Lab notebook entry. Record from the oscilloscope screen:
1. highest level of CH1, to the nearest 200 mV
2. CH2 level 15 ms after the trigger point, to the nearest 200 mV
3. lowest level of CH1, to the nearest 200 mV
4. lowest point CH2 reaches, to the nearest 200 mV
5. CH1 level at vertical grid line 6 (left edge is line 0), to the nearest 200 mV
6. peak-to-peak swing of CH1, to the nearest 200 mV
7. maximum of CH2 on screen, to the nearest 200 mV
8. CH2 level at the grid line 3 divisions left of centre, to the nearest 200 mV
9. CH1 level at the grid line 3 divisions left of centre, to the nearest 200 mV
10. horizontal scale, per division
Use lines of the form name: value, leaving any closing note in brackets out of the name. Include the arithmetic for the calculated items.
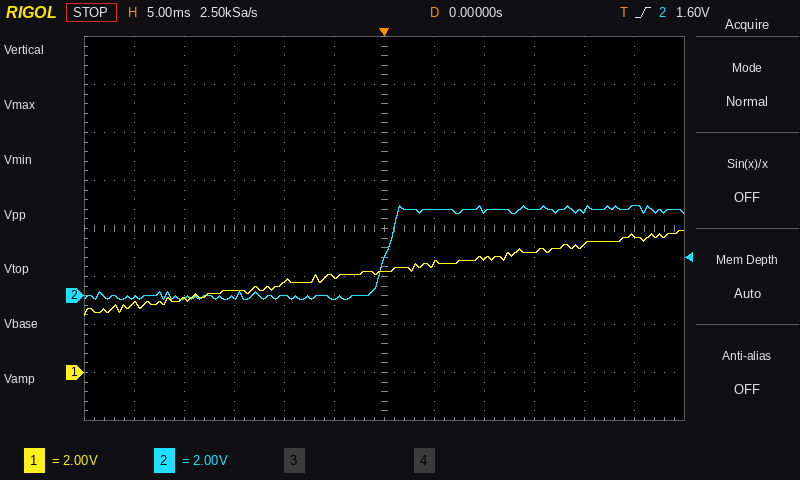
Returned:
highest level of CH1, to the nearest 200 mV: 6.0 V
CH2 level 15 ms after the trigger point, to the nearest 200 mV: 3.6 V
lowest level of CH1, to the nearest 200 mV: 2.4 V
lowest point CH2 reaches, to the nearest 200 mV: -200 mV
CH1 level at vertical grid line 6 (left edge is line 0), to the nearest 200 mV: 4.2 V
peak-to-peak swing of CH1, to the nearest 200 mV: 6.0 V − (2.4 V) = 3.6 V
maximum of CH2 on screen, to the nearest 200 mV: 3.8 V
CH2 level at the grid line 3 divisions left of centre, to the nearest 200 mV: 0.0 V
CH1 level at the grid line 3 divisions left of centre, to the nearest 200 mV: 3.4 V
horizontal scale, per division: 5 ms
